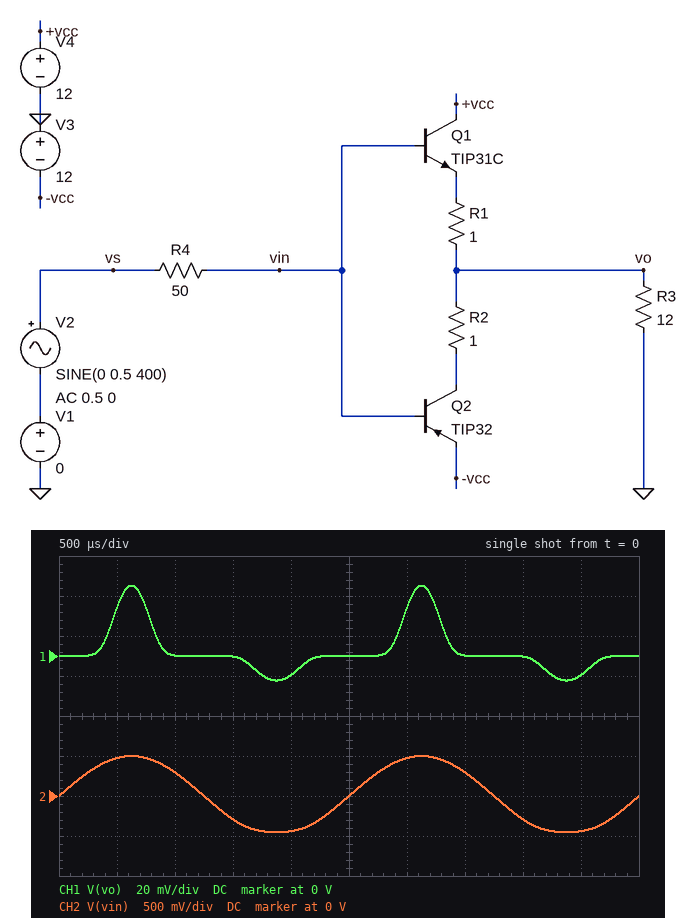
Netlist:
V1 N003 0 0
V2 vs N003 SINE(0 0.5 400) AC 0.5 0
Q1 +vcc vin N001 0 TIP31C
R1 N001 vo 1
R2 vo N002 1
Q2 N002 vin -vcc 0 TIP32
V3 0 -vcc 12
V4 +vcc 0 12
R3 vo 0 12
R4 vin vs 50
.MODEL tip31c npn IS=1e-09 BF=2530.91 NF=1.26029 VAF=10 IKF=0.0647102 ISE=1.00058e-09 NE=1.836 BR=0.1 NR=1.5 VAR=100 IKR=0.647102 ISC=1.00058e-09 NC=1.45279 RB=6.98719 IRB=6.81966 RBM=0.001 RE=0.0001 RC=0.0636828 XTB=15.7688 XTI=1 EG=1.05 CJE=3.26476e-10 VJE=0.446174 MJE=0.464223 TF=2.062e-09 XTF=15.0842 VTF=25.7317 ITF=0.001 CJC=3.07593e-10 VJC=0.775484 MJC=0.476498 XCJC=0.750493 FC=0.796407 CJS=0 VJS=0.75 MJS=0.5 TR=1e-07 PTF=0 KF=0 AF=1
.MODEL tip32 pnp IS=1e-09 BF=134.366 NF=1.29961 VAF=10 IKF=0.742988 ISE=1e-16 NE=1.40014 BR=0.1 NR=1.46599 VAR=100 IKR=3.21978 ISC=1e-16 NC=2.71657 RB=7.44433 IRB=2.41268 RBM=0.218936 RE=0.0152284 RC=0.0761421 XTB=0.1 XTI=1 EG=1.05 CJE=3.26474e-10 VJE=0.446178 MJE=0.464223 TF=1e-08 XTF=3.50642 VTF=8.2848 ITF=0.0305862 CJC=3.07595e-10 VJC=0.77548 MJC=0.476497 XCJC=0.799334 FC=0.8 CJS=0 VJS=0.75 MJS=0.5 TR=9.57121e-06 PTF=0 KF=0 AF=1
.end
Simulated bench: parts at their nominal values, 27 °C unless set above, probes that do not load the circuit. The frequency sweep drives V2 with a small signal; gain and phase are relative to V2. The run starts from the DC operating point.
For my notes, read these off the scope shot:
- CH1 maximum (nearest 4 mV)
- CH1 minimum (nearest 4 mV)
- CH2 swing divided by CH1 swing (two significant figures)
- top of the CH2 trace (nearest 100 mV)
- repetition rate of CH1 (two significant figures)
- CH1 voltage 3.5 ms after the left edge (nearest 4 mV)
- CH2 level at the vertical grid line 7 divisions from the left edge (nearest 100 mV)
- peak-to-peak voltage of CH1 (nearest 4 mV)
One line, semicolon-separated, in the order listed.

36 mV; -12 mV; 20; 500 mV; 400 Hz; 0 V; 300 mV; 48 mV
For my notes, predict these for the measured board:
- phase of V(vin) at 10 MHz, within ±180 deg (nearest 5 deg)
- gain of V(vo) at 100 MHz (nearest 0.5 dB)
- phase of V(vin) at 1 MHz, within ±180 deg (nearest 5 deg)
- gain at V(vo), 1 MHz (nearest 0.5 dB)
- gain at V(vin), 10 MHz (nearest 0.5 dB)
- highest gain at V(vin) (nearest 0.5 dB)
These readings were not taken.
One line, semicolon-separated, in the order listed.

-45 deg; -18.5 dB; -15 deg; -27.0 dB; -8.5 dB; 0 dB
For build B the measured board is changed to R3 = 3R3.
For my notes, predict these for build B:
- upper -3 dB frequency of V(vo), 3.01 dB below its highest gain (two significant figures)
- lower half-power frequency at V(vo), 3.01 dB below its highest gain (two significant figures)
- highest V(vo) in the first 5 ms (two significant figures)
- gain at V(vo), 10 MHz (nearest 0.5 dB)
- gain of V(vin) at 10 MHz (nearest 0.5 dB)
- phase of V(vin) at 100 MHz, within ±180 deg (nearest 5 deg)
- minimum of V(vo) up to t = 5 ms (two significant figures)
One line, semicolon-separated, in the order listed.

370 MHz; 3.6 MHz; 16 mV; -27.0 dB; -9.0 dB; -30 deg; -3.7 mV
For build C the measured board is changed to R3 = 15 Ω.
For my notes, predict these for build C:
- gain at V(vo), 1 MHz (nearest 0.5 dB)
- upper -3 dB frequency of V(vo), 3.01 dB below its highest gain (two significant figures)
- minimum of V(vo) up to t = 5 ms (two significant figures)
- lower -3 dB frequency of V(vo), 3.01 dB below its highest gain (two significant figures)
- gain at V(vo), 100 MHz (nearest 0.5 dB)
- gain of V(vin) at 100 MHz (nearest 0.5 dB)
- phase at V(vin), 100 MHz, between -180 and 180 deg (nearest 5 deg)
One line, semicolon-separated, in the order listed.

-25.0 dB; 110 MHz; -15 mV; 3.0 MHz; -17.5 dB; -15.0 dB; -40 deg
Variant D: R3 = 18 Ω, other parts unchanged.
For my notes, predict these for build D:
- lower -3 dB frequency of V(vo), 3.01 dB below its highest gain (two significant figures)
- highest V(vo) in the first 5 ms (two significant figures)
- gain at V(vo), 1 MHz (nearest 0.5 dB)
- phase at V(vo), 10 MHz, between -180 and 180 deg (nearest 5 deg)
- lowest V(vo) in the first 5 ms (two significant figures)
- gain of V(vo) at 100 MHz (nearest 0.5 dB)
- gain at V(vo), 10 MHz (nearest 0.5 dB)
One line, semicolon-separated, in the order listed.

2.9 MHz; 43 mV; -23.5 dB; 10 deg; -17 mV; -16.5 dB; -13.5 dB
